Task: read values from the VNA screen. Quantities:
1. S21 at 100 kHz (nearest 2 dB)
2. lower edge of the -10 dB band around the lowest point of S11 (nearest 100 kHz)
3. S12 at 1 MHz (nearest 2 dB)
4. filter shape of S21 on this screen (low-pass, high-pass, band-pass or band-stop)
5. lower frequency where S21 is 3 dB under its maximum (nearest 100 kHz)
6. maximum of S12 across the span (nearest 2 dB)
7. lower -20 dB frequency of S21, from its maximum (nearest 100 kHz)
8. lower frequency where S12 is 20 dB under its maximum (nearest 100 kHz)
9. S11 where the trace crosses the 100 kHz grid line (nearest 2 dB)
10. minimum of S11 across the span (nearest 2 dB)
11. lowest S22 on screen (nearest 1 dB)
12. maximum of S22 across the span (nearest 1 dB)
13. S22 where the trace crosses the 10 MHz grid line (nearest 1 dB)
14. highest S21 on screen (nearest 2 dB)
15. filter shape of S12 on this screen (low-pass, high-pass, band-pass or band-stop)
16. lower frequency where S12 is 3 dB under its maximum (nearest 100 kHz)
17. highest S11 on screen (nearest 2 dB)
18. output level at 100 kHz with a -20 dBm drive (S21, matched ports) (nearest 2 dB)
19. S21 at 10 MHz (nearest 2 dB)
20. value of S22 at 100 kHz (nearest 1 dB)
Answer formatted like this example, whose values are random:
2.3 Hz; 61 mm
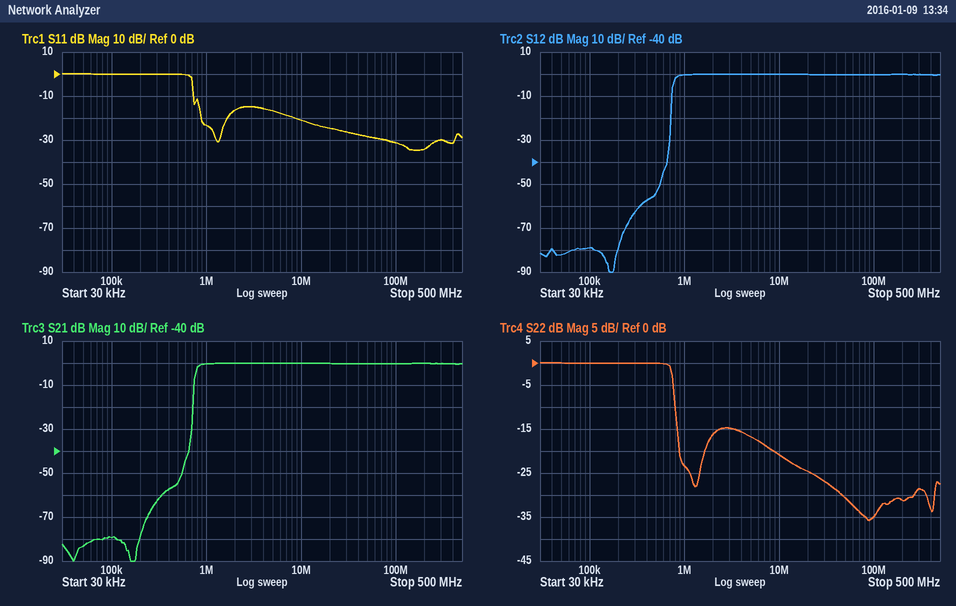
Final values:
-80 dB; 700 kHz; 0 dB; high-pass; 800 kHz; 0 dB; 700 kHz; 700 kHz; 0 dB; -34 dB; -36 dB; 0 dB; -21 dB; 0 dB; high-pass; 800 kHz; 0 dB; -100 dBm; 0 dB; 0 dB
